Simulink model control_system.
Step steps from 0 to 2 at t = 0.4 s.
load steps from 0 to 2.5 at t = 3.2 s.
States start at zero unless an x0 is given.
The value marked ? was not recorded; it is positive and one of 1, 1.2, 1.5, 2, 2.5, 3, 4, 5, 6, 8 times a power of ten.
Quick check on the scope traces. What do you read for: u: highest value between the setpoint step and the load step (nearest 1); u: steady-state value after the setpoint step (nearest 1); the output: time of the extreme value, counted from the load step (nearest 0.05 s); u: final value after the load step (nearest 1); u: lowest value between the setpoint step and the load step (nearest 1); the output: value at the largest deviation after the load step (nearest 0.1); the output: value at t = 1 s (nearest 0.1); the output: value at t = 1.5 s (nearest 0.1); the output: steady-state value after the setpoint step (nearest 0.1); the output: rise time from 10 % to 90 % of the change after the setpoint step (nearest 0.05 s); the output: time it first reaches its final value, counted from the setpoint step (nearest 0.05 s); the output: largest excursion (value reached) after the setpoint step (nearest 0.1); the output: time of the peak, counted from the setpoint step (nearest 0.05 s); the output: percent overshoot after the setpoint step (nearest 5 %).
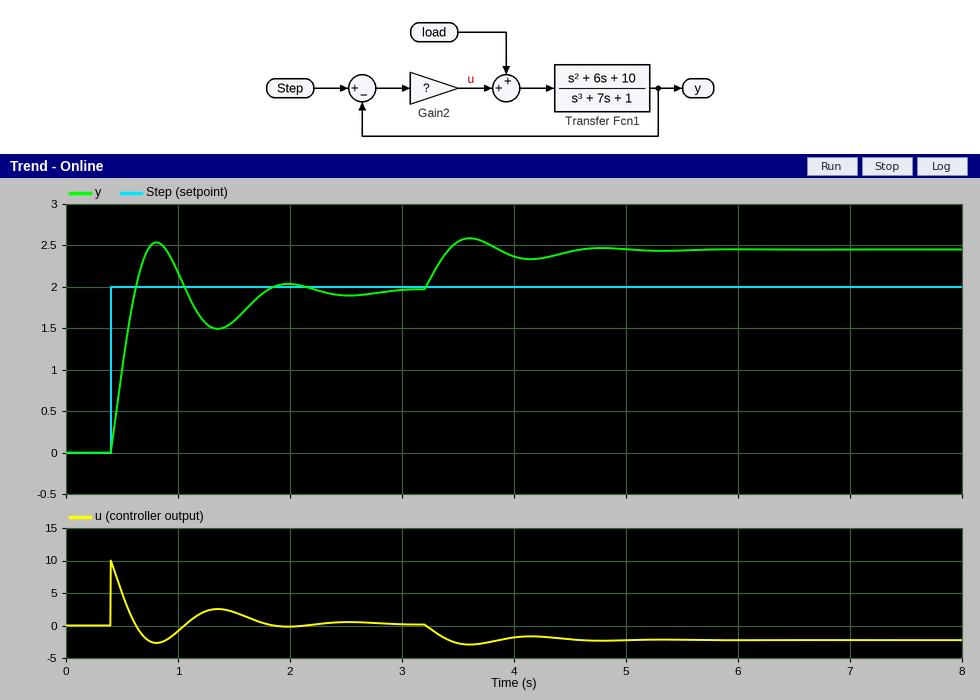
10
0
0.40 s
-2
-3
2.6
2.2
1.6
2.0
0.15 s
0.20 s
2.5
0.40 s
30 %
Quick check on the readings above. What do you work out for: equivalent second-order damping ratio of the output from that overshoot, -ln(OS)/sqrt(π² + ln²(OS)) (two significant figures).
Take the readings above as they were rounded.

0.36
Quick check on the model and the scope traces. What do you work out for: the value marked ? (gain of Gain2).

5
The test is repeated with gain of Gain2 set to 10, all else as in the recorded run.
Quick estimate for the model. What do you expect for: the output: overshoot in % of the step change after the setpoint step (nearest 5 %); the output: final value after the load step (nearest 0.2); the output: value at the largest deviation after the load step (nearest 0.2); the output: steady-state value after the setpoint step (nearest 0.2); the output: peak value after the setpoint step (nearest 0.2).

25 %
2.2
2.2
2.0
2.4
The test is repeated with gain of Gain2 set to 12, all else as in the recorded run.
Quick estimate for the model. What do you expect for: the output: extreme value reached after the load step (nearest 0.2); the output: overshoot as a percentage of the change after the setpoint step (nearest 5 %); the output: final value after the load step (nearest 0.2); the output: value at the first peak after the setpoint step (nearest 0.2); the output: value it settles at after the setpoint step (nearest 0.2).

2.2
20 %
2.2
2.4
2.0
